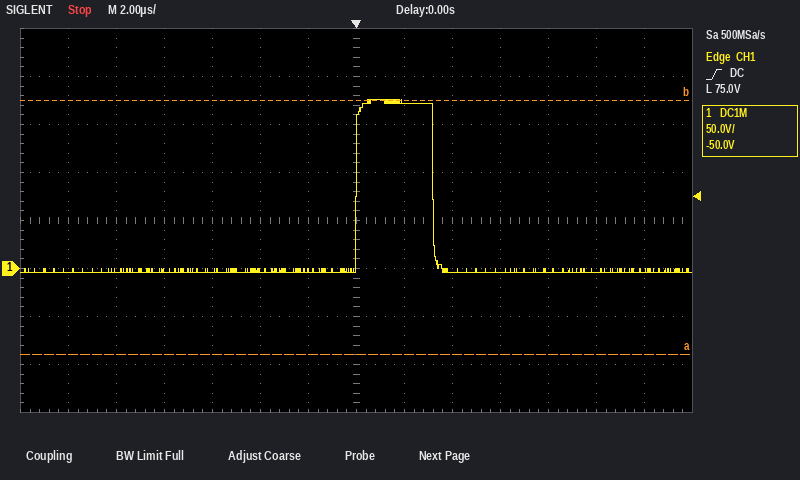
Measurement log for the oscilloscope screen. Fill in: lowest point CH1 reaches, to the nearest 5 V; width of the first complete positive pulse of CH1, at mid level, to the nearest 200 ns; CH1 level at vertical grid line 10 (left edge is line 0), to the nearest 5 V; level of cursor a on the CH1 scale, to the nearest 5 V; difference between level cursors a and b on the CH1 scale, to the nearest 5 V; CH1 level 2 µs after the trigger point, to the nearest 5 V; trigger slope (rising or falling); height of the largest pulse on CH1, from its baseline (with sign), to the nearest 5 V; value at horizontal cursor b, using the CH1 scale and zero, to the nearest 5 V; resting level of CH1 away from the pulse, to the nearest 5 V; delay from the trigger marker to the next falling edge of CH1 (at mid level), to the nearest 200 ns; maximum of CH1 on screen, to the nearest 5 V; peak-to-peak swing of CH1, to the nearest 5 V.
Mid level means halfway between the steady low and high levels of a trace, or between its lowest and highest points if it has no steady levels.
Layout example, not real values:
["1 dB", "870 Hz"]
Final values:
["-5 V", "3.2 µs", "-5 V", "-90 V", "265 V", "170 V", "rising", "+180 V", "175 V", "-5 V", "3.2 µs", "175 V", "180 V"]
